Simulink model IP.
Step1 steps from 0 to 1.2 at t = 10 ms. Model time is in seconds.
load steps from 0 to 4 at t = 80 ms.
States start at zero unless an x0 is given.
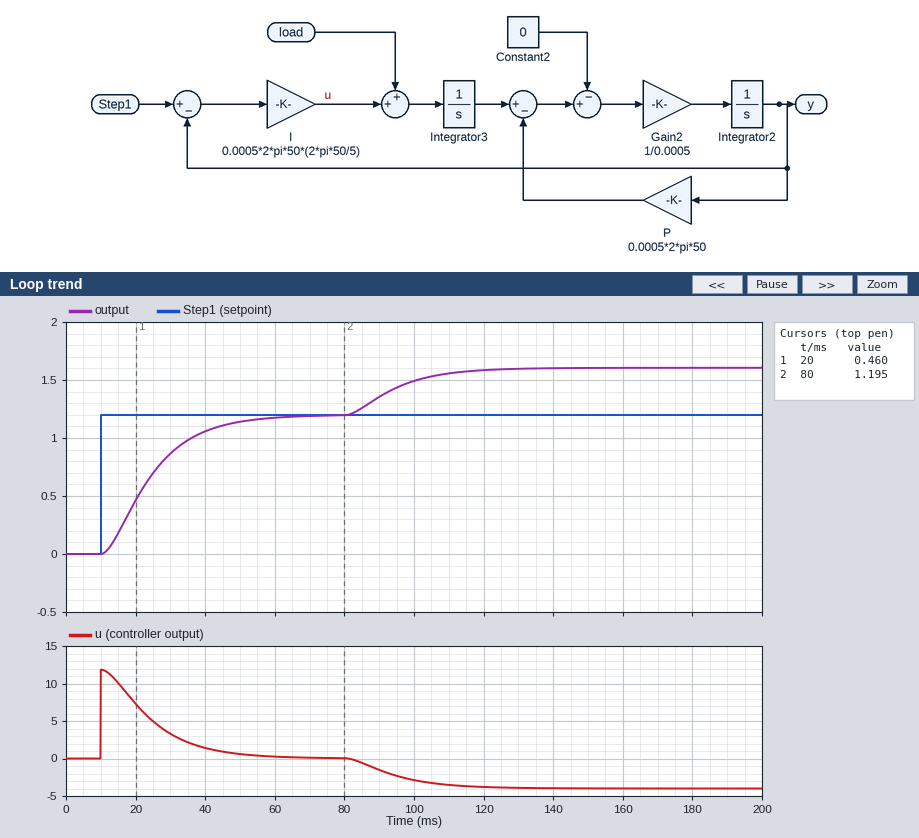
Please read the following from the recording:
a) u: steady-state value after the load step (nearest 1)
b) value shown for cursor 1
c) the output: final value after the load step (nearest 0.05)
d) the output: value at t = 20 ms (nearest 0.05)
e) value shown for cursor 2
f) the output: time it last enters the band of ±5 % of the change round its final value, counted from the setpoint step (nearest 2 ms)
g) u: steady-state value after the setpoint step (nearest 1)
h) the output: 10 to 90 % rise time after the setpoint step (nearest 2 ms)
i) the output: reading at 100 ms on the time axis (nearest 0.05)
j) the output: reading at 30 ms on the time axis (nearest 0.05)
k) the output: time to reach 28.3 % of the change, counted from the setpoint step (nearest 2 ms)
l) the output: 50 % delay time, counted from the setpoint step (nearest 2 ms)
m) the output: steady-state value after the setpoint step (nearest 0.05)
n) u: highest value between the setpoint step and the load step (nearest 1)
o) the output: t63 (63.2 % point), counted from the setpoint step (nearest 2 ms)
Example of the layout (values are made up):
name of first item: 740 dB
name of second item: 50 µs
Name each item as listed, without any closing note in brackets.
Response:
u: steady-state value after the load step: -4
value shown for cursor 1: 0.460
the output: final value after the load step: 1.60
the output: value at t = 20 ms: 0.45
value shown for cursor 2: 1.195
the output: time it last enters the band of ±5 % of the change round its final value, counted from the setpoint step: 40 ms
u: steady-state value after the setpoint step: 0
the output: 10 to 90 % rise time after the setpoint step: 28 ms
the output: reading at 100 ms on the time axis: 1.50
the output: reading at 30 ms on the time axis: 0.85
the output: time to reach 28.3 % of the change, counted from the setpoint step: 8 ms
the output: 50 % delay time, counted from the setpoint step: 12 ms
the output: steady-state value after the setpoint step: 1.20
u: highest value between the setpoint step and the load step: 12
the output: t63 (63.2 % point), counted from the setpoint step: 16 ms
